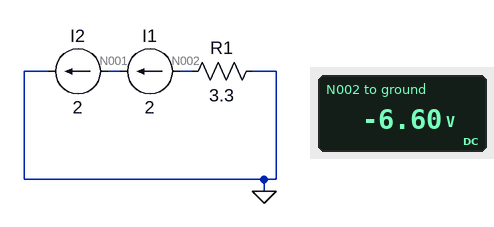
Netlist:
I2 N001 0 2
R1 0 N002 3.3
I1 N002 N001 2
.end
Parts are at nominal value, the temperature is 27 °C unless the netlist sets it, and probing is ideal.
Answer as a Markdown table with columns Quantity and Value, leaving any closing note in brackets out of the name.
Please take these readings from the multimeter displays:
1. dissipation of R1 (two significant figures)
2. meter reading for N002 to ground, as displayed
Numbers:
| Quantity | Value |
|---|---|
| dissipation of R1 | 13 W |
| meter reading for N002 to ground, as displayed | -6.60 V |
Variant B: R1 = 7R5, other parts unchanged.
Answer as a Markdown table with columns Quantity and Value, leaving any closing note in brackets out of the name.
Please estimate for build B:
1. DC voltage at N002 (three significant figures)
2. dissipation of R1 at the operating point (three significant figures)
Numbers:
| Quantity | Value |
|---|---|
| DC voltage at N002 | -15.0 V |
| dissipation of R1 at the operating point | 30.0 W |
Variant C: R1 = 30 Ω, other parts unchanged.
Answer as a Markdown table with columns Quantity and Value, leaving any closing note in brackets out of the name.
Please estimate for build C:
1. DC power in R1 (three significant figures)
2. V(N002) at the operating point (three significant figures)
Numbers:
| Quantity | Value |
|---|---|
| DC power in R1 | 120 W |
| V(N002) at the operating point | -60.0 V |
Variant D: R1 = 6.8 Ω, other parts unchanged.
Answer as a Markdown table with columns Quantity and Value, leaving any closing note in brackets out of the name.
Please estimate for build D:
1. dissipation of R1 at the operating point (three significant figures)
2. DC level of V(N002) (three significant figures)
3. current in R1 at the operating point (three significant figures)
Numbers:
| Quantity | Value |
|---|---|
| dissipation of R1 at the operating point | 27.2 W |
| DC level of V(N002) | -13.6 V |
| current in R1 at the operating point | 2.00 A |
